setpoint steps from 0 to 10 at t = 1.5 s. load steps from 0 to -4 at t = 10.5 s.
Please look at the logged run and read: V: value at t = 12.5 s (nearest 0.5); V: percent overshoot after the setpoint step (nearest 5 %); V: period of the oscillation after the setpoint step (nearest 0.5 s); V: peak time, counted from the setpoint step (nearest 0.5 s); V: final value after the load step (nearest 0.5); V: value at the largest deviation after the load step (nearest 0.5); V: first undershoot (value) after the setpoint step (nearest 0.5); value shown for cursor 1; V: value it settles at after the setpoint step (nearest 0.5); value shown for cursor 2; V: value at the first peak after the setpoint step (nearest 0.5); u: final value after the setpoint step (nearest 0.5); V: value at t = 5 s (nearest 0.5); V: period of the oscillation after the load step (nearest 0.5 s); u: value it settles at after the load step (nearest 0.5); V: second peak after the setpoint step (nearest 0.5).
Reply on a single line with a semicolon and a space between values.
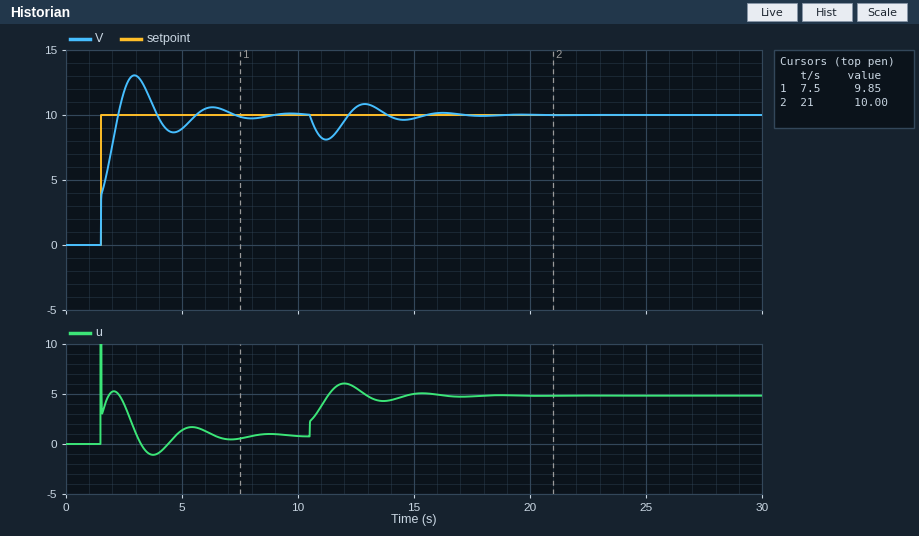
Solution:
10.5; 30 %; 3.5 s; 1.5 s; 10.0; 8.0; 8.5; 9.85; 10.0; 10.00; 13.0; 1.0; 9.0; 3.5 s; 5.0; 10.5
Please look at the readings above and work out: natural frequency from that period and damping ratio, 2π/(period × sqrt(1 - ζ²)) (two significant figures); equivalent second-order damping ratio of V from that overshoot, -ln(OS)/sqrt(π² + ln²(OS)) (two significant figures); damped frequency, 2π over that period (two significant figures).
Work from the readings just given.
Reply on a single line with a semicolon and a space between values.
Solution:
1.9 rad/s; 0.36; 1.8 rad/s
